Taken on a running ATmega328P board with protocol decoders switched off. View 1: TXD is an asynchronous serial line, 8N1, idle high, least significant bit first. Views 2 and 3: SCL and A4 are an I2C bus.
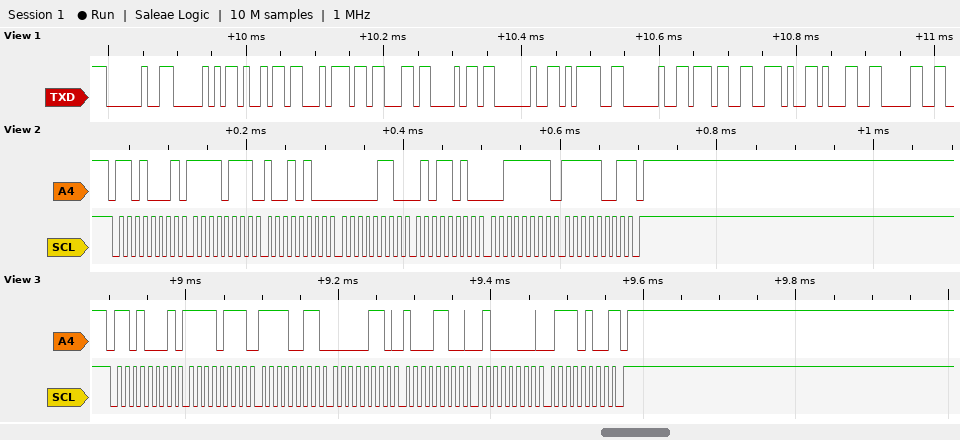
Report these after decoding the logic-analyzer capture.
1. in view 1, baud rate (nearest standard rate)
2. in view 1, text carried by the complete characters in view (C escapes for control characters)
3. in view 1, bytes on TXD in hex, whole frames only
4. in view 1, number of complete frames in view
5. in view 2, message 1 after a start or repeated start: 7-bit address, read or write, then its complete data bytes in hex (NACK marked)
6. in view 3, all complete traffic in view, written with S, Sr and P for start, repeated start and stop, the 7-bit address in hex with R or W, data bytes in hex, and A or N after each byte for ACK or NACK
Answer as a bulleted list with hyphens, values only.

- 115200 baud
- " Pitch = 7.10"
- 20 50 69 74 63 68 20 3D 20 37 2E 31 30
- 13
- 0x68 read: F7 94 06 5A 3F F9 NACK
- S 68R A F7 A F3 A 06 A 8C A 40 A 74 N P
